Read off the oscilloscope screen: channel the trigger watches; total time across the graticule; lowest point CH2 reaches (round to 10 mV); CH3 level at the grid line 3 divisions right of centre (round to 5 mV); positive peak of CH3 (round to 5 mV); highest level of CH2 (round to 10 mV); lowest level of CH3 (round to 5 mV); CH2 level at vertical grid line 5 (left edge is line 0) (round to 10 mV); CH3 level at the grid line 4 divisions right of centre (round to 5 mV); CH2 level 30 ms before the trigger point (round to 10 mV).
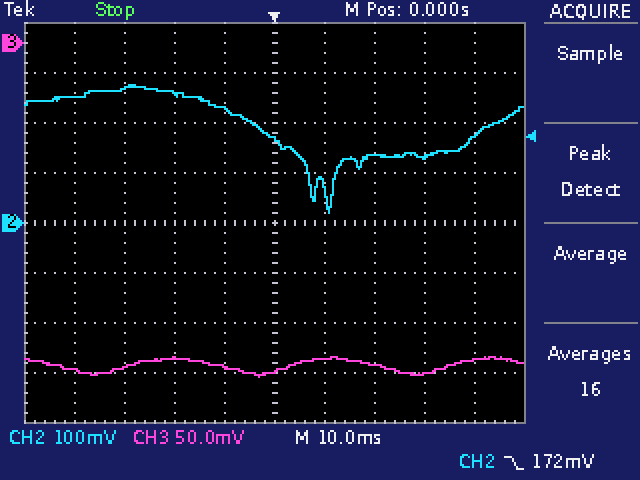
CH2
100 ms
20 mV
-330 mV
-315 mV
280 mV
-335 mV
170 mV
-315 mV
270 mV
